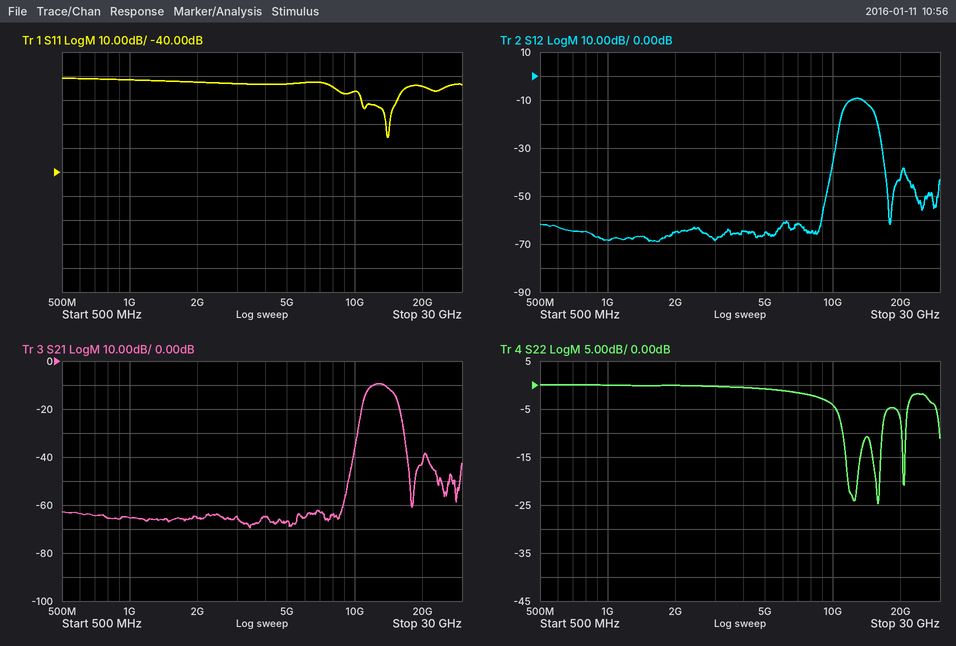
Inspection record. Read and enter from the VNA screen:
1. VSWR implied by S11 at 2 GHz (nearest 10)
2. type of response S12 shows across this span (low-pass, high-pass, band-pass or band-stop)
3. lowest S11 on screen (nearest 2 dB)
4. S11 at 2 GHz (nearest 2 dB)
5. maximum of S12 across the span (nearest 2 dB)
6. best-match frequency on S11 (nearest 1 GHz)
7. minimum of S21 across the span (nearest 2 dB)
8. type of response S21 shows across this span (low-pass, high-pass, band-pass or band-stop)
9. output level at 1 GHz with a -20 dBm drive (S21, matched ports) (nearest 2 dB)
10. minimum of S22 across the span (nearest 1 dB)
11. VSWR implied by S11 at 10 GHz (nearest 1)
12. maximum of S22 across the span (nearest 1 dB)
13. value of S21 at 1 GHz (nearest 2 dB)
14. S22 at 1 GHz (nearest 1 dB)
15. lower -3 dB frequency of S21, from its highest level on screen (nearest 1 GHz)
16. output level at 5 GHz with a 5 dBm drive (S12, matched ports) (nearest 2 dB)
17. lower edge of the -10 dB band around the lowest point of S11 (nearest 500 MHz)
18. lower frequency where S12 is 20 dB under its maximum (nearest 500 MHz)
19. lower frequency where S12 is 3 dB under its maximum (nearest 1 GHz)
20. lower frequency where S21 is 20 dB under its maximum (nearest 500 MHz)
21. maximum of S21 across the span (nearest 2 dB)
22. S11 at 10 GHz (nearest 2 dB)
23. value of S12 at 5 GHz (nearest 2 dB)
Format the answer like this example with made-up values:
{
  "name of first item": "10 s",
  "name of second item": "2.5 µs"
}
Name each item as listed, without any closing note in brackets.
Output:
{
  "VSWR implied by S11 at 2 GHz": "10",
  "type of response S12 shows across this span": "band-pass",
  "lowest S11 on screen": "-26 dB",
  "S11 at 2 GHz": "-2 dB",
  "maximum of S12 across the span": "-10 dB",
  "best-match frequency on S11": "14 GHz",
  "minimum of S21 across the span": "-70 dB",
  "type of response S21 shows across this span": "band-pass",
  "output level at 1 GHz with a -20 dBm drive (S21, matched ports)": "-86 dBm",
  "minimum of S22 across the span": "-25 dB",
  "VSWR implied by S11 at 10 GHz": "3",
  "maximum of S22 across the span": "0 dB",
  "value of S21 at 1 GHz": "-66 dB",
  "S22 at 1 GHz": "0 dB",
  "lower -3 dB frequency of S21, from its highest level on screen": "11 GHz",
  "output level at 5 GHz with a 5 dBm drive (S12, matched ports)": "-60 dBm",
  "lower edge of the -10 dB band around the lowest point of S11": "10.5 GHz",
  "lower frequency where S12 is 20 dB under its maximum": "10.5 GHz",
  "lower frequency where S12 is 3 dB under its maximum": "11 GHz",
  "lower frequency where S21 is 20 dB under its maximum": "10.5 GHz",
  "maximum of S21 across the span": "-10 dB",
  "S11 at 10 GHz": "-6 dB",
  "value of S12 at 5 GHz": "-66 dB"
}
